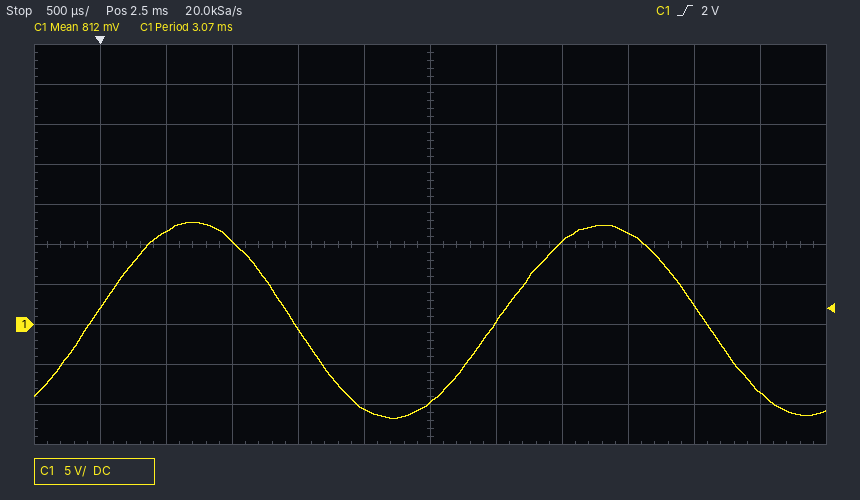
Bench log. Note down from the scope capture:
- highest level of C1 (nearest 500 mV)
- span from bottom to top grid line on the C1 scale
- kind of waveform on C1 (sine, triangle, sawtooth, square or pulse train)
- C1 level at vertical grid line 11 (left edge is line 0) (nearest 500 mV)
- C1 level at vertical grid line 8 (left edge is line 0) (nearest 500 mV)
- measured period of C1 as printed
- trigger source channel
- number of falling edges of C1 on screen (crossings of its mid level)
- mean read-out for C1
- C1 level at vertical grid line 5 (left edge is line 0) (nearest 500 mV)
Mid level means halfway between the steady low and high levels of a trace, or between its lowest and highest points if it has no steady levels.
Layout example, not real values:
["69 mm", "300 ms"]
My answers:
["13.0 V", "50 V", "sine", "-8.5 V", "10.5 V", "3.07 ms", "C1", "2", "812 mV", "-10.5 V"]
